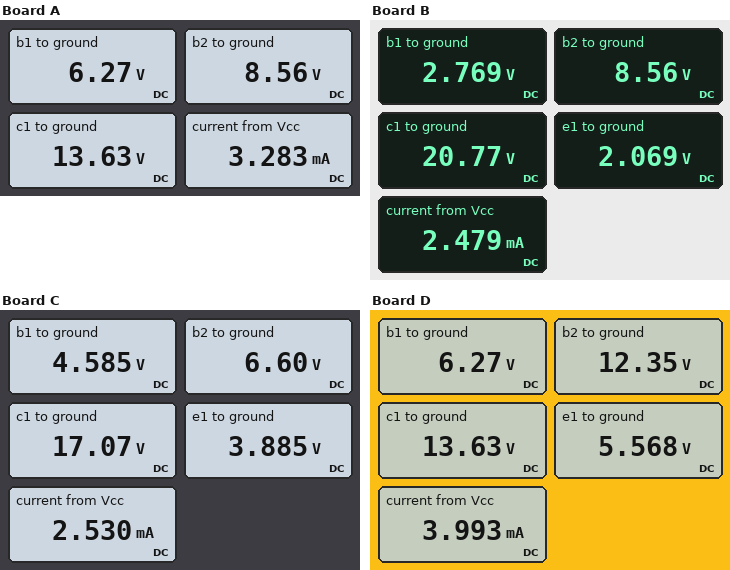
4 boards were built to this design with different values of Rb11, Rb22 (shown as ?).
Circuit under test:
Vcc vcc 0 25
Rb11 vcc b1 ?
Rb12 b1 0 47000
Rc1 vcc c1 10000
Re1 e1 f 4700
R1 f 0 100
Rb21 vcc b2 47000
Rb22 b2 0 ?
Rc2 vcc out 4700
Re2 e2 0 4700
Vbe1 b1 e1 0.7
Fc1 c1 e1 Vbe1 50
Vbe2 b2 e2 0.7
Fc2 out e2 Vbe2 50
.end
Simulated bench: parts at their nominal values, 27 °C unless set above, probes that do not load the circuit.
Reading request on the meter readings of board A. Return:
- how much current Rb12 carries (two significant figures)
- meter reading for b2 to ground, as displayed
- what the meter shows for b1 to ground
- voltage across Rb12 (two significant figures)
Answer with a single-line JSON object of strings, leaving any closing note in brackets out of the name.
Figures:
{"how much current Rb12 carries": "130 µA", "meter reading for b2 to ground, as displayed": "8.56 V", "what the meter shows for b1 to ground": "6.27 V", "voltage across Rb12": "6.3 V"}
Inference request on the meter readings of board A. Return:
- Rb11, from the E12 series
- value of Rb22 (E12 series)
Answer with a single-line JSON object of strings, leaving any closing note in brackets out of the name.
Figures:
{"Rb11, from the E12 series": "120 kΩ", "value of Rb22": "27 kΩ"}
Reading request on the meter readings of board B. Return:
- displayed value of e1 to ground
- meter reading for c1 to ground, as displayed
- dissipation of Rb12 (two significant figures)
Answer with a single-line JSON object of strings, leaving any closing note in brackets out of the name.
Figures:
{"displayed value of e1 to ground": "2.069 V", "meter reading for c1 to ground, as displayed": "20.77 V", "dissipation of Rb12": "160 µW"}
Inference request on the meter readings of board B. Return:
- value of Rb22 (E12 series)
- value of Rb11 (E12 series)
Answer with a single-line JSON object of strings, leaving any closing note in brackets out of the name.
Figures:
{"value of Rb22": "27 kΩ", "value of Rb11": "330 kΩ"}
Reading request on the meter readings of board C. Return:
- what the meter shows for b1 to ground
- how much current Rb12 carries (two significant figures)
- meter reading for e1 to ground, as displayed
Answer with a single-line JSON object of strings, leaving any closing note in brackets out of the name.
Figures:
{"what the meter shows for b1 to ground": "4.585 V", "how much current Rb12 carries": "98 µA", "meter reading for e1 to ground, as displayed": "3.885 V"}
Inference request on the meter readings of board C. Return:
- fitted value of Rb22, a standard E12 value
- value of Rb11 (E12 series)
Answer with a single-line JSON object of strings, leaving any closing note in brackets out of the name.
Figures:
{"fitted value of Rb22, a standard E12 value": "18 kΩ", "value of Rb11": "180 kΩ"}
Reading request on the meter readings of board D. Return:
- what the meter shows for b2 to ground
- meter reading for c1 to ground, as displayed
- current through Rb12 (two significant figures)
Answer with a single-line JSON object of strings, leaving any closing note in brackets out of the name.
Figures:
{"what the meter shows for b2 to ground": "12.35 V", "meter reading for c1 to ground, as displayed": "13.63 V", "current through Rb12": "130 µA"}
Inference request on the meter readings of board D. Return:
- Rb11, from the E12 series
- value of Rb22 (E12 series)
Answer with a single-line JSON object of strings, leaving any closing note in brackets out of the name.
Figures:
{"Rb11, from the E12 series": "120 kΩ", "value of Rb22": "56 kΩ"}
